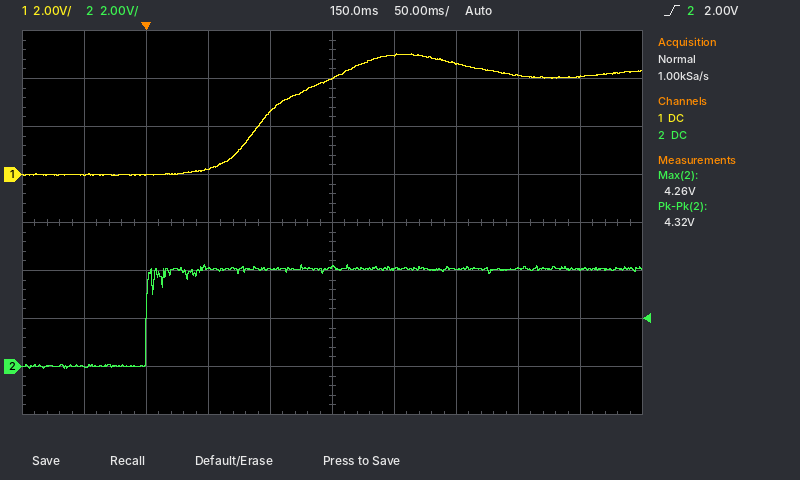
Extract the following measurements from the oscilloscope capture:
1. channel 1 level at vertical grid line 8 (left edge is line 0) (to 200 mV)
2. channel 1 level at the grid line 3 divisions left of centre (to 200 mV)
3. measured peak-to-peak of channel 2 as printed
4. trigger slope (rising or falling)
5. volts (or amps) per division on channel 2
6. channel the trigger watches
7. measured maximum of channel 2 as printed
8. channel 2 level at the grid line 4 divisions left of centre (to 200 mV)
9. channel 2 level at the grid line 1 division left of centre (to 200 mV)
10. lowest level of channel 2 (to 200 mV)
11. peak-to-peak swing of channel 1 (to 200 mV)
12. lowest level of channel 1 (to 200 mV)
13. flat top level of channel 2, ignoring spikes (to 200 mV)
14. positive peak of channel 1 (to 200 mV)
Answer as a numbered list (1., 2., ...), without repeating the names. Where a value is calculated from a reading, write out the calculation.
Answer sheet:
1. 4.2 V
2. 0.0 V
3. 4.32 V
4. rising
5. 2 V
6. channel 2
7. 4.26 V
8. 0.0 V
9. 4.0 V
10. 0.0 V
11. 5.0 V − (0.0 V) = 5.0 V
12. 0.0 V
13. 4.0 V
14. 5.0 V
